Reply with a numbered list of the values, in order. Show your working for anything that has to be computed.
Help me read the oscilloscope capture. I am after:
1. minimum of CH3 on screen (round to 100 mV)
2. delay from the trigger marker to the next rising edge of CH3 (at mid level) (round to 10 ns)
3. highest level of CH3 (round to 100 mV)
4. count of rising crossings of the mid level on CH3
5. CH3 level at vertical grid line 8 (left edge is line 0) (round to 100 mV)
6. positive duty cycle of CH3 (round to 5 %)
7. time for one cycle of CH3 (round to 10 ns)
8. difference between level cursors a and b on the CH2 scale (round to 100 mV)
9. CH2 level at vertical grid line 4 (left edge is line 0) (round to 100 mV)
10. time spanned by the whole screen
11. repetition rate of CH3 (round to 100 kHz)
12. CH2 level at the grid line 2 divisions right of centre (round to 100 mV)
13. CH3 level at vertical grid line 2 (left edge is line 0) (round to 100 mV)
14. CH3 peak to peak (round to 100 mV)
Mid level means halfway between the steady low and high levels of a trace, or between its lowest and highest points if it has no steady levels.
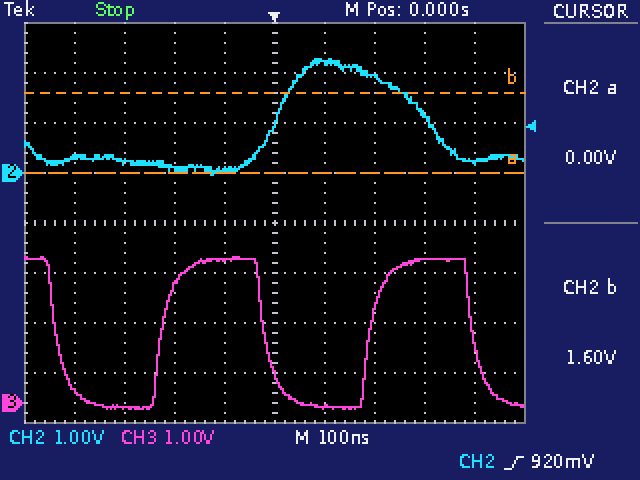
1. -100 mV
2. 190 ns
3. 2.9 V
4. 2
5. 2.9 V
6. 50 %
7. 420 ns
8. 1.6 V
9. 100 mV
10. 1 µs
11. 1 / 420 ns ≈ 2.4 MHz
12. 1.9 V
13. -100 mV
14. 2.9 V − (-100 mV) = 3.0 V
